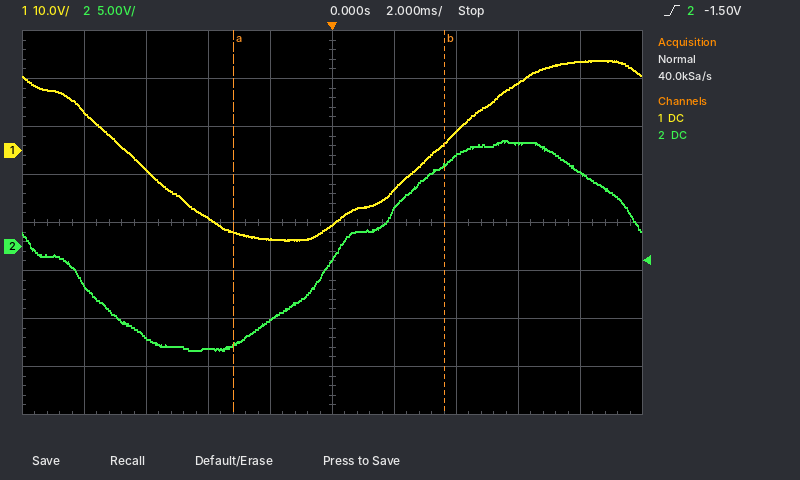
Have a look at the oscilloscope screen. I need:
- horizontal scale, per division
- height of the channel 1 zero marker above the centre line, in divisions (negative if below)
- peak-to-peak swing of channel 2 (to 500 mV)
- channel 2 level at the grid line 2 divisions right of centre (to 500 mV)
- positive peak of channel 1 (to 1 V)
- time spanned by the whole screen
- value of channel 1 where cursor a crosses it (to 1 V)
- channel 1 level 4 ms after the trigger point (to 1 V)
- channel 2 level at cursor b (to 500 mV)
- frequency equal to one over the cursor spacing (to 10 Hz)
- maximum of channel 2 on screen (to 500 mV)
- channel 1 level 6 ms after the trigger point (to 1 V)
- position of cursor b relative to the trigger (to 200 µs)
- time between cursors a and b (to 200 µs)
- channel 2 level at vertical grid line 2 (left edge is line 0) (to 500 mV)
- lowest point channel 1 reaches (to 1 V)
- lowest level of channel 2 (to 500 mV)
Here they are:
2 ms
+1.5 div
22.0 V
9.5 V
19 V
20 ms
-17 V
4 V
8.5 V
150 Hz
11.0 V
14 V
+3.6 ms
6.8 ms
-9.5 V
-19 V
-11.0 V
